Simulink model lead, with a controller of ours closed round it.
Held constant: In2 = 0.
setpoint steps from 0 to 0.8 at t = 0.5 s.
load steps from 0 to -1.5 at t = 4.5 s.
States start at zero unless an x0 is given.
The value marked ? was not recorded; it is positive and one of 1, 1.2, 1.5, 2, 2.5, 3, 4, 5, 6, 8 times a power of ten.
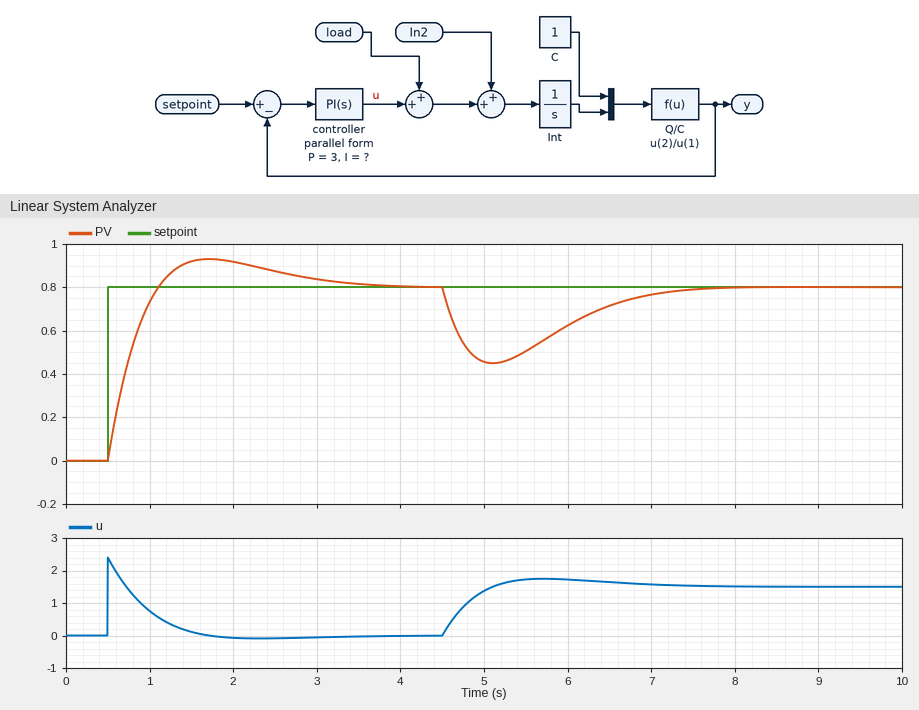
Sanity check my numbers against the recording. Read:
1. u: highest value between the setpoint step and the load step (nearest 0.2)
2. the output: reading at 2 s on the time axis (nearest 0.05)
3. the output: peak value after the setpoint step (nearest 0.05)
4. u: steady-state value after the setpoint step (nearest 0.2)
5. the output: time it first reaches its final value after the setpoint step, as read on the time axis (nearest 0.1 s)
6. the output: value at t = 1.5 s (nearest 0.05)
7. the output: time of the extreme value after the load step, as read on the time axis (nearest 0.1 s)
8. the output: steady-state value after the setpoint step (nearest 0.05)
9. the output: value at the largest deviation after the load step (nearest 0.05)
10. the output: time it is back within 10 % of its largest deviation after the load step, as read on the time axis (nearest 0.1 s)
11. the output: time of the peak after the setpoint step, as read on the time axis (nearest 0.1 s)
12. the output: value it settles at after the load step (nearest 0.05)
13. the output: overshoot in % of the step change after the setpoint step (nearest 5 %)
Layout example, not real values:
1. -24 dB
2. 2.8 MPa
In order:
1. 2.4
2. 0.90
3. 0.95
4. 0.0
5. 1.1 s
6. 0.90
7. 5.1 s
8. 0.80
9. 0.45
10. 7.0 s
11. 1.7 s
12. 0.80
13. 15 %
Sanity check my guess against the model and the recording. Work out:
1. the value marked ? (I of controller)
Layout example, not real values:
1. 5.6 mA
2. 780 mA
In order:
1. 3
